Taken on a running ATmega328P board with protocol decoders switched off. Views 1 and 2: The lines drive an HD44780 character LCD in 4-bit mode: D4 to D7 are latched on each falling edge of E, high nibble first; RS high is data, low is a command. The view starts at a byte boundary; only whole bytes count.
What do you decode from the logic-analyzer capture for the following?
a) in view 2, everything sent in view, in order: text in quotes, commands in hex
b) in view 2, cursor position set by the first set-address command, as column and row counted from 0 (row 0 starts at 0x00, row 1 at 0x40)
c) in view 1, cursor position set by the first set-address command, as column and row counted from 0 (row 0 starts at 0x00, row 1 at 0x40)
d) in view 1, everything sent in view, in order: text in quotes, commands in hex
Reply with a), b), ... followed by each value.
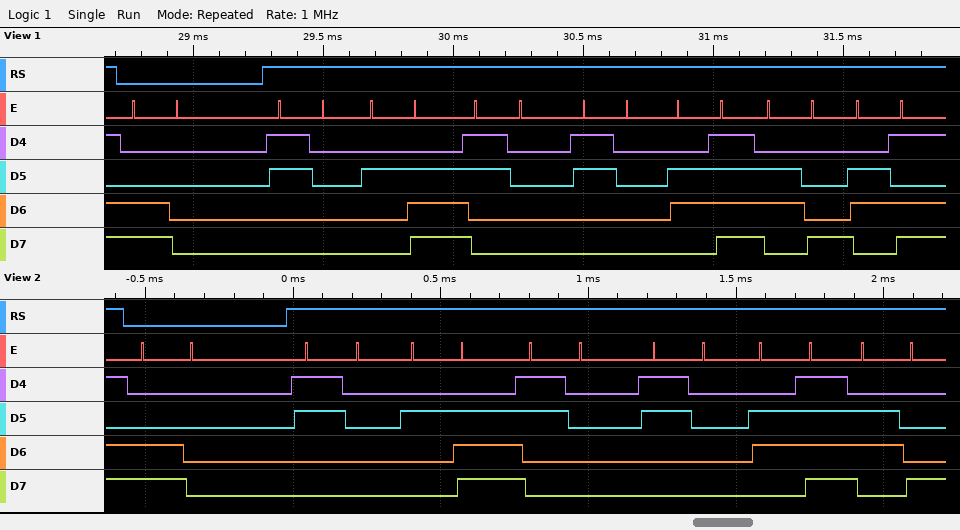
a) 0xC0 "0.00oh"
b) column 0, row 1
c) column 0, row 1
d) 0xC0 "0.00ohm"
